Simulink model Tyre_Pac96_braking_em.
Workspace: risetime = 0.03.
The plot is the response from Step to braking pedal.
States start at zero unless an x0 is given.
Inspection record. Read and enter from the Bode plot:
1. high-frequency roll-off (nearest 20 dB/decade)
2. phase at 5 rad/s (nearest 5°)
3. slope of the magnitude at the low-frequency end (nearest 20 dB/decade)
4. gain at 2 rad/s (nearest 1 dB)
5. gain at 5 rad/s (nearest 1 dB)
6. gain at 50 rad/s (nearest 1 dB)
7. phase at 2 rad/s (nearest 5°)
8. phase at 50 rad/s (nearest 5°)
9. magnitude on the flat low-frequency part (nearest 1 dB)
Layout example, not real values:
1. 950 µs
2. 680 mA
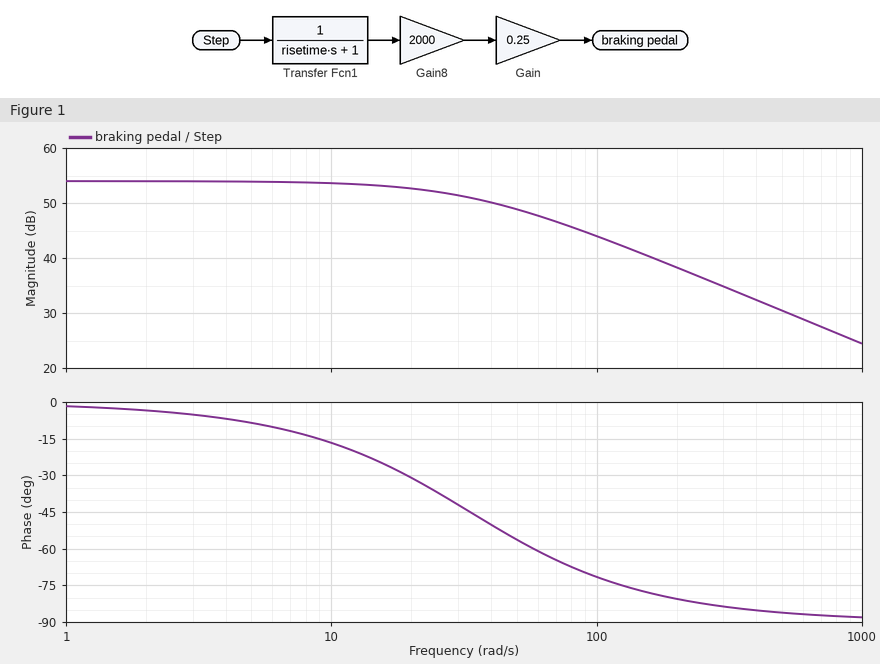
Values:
1. -20 dB/decade
2. -10°
3. 0 dB/decade
4. 54 dB
5. 54 dB
6. 49 dB
7. -5°
8. -55°
9. 54 dB
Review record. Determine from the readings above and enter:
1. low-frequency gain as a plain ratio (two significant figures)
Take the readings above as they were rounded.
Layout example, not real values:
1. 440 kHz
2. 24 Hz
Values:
1. 500
